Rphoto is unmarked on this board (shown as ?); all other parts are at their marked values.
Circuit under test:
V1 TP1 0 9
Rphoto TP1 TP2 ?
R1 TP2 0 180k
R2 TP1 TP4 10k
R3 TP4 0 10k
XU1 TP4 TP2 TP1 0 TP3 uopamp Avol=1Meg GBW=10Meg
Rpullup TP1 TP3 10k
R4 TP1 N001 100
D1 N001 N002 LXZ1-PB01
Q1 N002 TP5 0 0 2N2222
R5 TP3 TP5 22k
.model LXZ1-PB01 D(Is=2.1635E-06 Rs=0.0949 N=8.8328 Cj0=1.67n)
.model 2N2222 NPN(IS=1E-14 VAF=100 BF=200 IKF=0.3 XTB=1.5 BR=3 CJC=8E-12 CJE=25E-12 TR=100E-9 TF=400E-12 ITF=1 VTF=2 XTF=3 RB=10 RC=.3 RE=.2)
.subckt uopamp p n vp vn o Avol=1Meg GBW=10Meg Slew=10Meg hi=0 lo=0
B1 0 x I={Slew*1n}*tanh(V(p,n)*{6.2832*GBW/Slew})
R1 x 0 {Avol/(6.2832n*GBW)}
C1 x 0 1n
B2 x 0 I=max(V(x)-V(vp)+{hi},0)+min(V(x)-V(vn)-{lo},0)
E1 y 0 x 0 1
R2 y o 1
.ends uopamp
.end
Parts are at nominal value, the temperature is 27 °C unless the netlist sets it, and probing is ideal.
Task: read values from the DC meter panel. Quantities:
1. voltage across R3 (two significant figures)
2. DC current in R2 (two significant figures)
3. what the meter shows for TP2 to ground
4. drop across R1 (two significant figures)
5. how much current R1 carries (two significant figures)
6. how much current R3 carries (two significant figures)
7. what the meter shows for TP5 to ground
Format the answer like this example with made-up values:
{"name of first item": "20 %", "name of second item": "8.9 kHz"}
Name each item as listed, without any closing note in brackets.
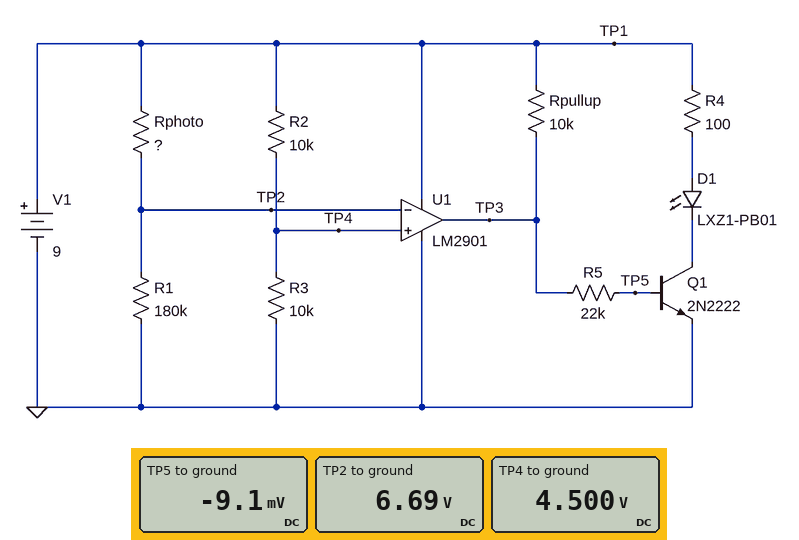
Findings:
{"voltage across R3": "4.5 V", "DC current in R2": "450 µA", "what the meter shows for TP2 to ground": "6.69 V", "drop across R1": "6.7 V", "how much current R1 carries": "37 µA", "how much current R3 carries": "450 µA", "what the meter shows for TP5 to ground": "-9.1 mV"}
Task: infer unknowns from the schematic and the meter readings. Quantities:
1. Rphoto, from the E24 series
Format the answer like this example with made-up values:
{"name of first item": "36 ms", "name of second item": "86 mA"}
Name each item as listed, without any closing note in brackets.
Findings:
{"Rphoto, from the E24 series": "62 kΩ"}
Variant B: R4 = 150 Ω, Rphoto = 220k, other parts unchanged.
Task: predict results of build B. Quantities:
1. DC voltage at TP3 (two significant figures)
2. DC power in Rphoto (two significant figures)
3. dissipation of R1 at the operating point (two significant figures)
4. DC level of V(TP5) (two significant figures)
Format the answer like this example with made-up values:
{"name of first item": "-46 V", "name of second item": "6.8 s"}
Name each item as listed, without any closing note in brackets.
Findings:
{"DC voltage at TP3": "9.0 V", "DC power in Rphoto": "110 µW", "dissipation of R1 at the operating point": "91 µW", "DC level of V(TP5)": "770 mV"}
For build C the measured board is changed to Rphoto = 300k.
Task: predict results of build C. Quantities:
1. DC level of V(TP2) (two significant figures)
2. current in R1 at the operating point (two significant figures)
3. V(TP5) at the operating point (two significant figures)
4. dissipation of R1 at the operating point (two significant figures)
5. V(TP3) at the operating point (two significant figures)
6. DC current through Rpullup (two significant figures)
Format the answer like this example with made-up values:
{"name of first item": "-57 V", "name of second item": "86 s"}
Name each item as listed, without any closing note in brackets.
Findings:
{"DC level of V(TP2)": "3.4 V", "current in R1 at the operating point": "19 µA", "V(TP5) at the operating point": "780 mV", "dissipation of R1 at the operating point": "63 µW", "V(TP3) at the operating point": "9.0 V", "DC current through Rpullup": "960 nA"}
